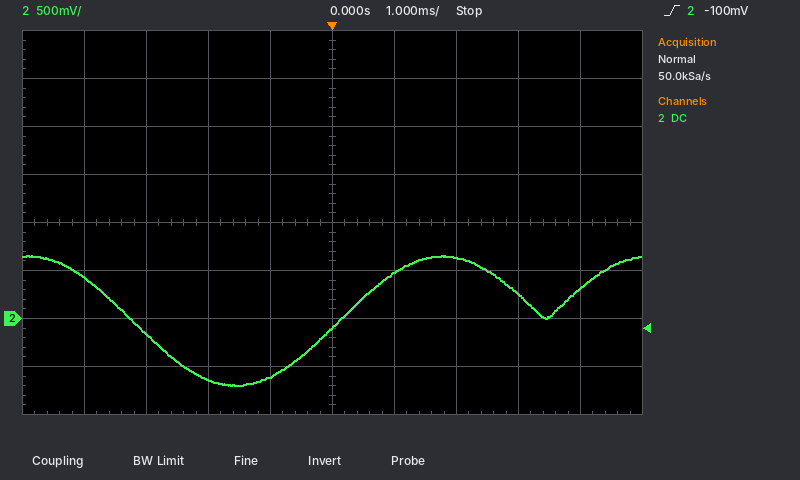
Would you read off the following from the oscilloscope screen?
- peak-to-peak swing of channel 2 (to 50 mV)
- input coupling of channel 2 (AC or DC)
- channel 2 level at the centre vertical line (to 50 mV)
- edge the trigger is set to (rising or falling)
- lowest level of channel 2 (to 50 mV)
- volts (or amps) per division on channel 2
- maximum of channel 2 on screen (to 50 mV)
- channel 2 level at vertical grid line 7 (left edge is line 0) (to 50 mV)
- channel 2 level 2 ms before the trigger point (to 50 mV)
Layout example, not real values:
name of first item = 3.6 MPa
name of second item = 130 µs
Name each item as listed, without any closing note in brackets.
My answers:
peak-to-peak swing of channel 2 = 1.35 V
input coupling of channel 2 = DC
channel 2 level at the centre vertical line = -100 mV
edge the trigger is set to = rising
lowest level of channel 2 = -700 mV
volts (or amps) per division on channel 2 = 500 mV
maximum of channel 2 on screen = 650 mV
channel 2 level at vertical grid line 7 (left edge is line 0) = 650 mV
channel 2 level 2 ms before the trigger point = -650 mV
